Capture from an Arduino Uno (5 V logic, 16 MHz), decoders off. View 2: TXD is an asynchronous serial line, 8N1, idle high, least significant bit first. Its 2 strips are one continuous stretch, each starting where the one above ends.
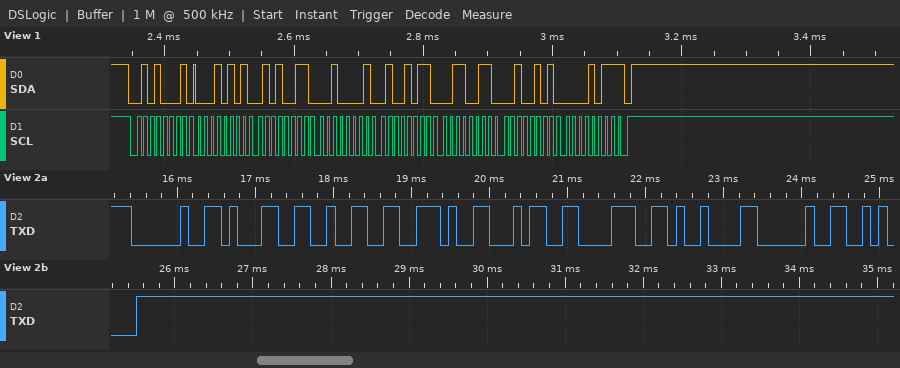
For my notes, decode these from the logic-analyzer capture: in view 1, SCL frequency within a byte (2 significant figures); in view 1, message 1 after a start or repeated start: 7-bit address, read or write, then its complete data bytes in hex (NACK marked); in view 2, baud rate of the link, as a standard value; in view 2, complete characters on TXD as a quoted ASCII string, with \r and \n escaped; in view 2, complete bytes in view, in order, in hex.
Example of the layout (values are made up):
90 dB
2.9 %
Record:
100 kHz
0x28 read: 15 53 21 4B 33 25 0B NACK
9600 baud
" 12.48\t \n"
20 31 32 2E 34 38 09 20 0A
